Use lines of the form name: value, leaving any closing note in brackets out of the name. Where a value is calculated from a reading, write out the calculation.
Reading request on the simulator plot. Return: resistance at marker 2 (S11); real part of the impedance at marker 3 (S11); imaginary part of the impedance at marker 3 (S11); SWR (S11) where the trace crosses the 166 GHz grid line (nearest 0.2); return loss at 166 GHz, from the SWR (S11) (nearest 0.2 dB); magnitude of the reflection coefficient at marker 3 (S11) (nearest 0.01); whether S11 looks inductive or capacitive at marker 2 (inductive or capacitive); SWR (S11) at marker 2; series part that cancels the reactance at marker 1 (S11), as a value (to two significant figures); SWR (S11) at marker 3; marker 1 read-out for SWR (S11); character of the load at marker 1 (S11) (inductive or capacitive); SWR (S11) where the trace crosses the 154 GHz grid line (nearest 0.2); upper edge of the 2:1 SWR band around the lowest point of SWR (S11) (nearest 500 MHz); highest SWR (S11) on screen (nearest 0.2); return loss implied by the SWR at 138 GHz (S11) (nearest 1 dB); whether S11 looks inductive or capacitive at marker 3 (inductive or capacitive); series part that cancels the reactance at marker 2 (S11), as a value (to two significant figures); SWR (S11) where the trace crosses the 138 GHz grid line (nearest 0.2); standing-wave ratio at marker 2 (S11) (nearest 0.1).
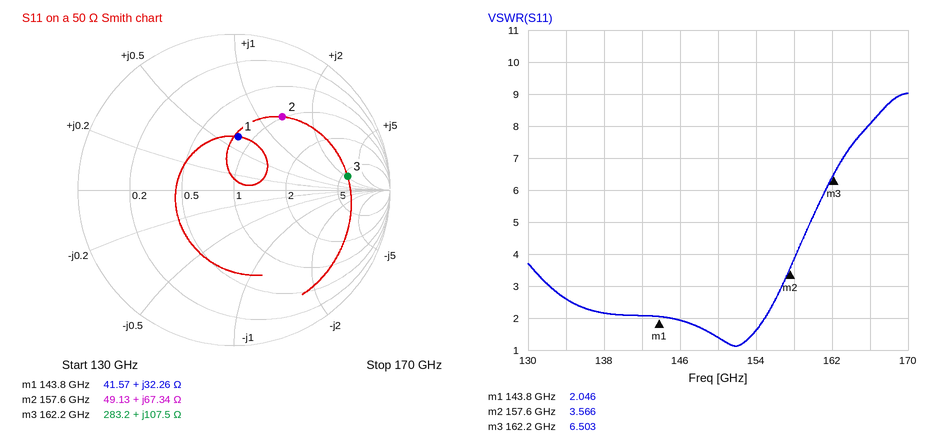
resistance at marker 2: 49.13 Ω
real part of the impedance at marker 3: 283.2 Ω
imaginary part of the impedance at marker 3: +107.5 Ω
SWR (S11) where the trace crosses the 166 GHz grid line: 8.0
return loss at 166 GHz, from the SWR (S11): −20 log10((8 − 1)/(8 + 1)) ≈ 2.2 dB
magnitude of the reflection coefficient at marker 3 (S11): 0.73
whether S11 looks inductive or capacitive at marker 2: inductive
SWR (S11) at marker 2: 3.566
series part that cancels the reactance at marker 1 (S11), as a value: C = 1/(2π × 143.8 GHz × 32.26 Ω) ≈ 34 fF
SWR (S11) at marker 3: 6.503
marker 1 read-out for SWR: 2.046
character of the load at marker 1 (S11): inductive
SWR (S11) where the trace crosses the 154 GHz grid line: 1.6
upper edge of the 2:1 SWR band around the lowest point of SWR (S11): 155.0 GHz
highest SWR (S11) on screen: 9.0
return loss implied by the SWR at 138 GHz (S11): −20 log10((2.2 − 1)/(2.2 + 1)) ≈ 9 dB
whether S11 looks inductive or capacitive at marker 3: inductive
series part that cancels the reactance at marker 2 (S11), as a value: C = 1/(2π × 157.6 GHz × 67.34 Ω) ≈ 15 fF
SWR (S11) where the trace crosses the 138 GHz grid line: 2.2
standing-wave ratio at marker 2 (S11): 3.6
